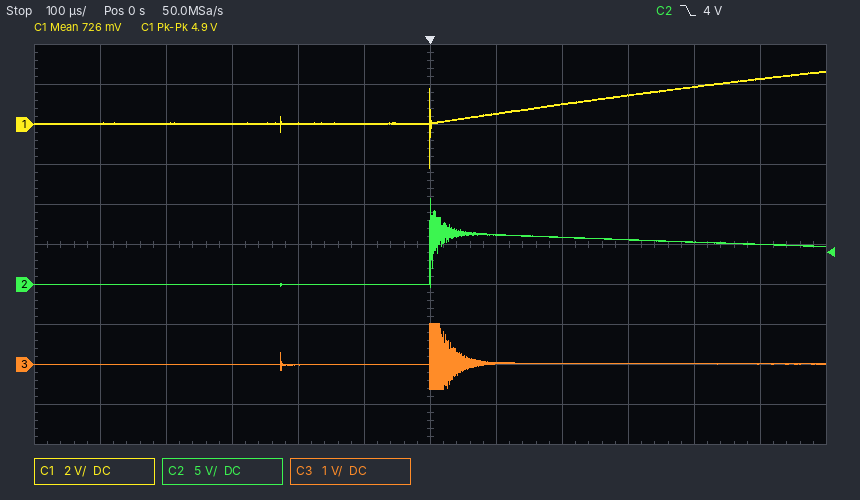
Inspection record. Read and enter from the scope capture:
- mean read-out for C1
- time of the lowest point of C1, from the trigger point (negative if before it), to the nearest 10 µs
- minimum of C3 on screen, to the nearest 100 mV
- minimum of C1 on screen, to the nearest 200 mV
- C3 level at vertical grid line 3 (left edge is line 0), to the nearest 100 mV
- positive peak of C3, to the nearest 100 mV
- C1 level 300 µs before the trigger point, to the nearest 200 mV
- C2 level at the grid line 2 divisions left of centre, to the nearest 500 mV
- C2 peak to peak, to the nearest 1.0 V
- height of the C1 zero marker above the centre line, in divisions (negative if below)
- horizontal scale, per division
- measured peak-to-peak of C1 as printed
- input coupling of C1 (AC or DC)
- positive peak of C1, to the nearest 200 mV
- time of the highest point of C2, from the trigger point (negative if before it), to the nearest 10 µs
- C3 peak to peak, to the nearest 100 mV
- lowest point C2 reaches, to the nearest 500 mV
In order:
726 mV
0 µs
-600 mV
-2.2 V
0.0 V
1.0 V
0.0 V
0.0 V
11.0 V
+3.0 div
100 µs
4.9 V
DC
2.6 V
0 µs
1.6 V
-500 mV
